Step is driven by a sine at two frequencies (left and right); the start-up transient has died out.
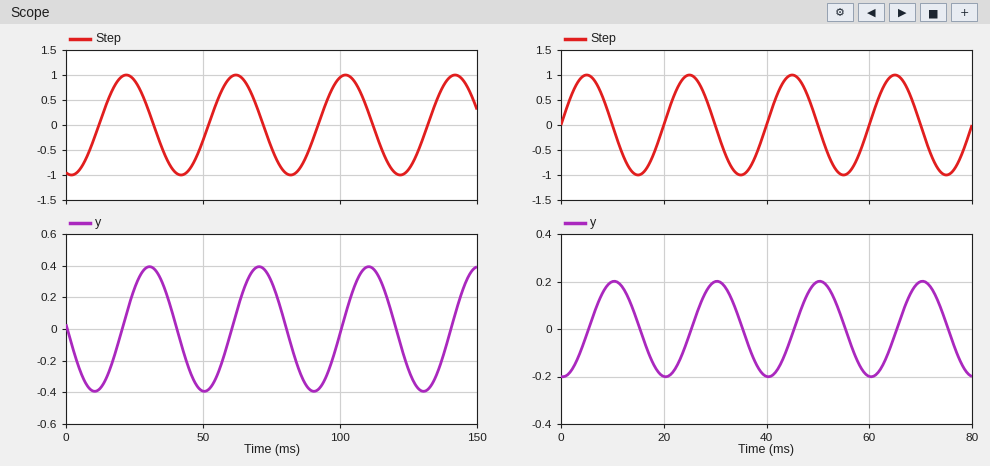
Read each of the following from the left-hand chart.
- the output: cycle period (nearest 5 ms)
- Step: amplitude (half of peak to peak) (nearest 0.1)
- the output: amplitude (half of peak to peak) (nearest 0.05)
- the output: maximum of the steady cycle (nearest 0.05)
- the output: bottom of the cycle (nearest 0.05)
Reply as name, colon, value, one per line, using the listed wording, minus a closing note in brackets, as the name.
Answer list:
the output: cycle period: 40 ms
Step: amplitude (half of peak to peak): 1.0
the output: amplitude (half of peak to peak): 0.40
the output: maximum of the steady cycle: 0.40
the output: bottom of the cycle: -0.40
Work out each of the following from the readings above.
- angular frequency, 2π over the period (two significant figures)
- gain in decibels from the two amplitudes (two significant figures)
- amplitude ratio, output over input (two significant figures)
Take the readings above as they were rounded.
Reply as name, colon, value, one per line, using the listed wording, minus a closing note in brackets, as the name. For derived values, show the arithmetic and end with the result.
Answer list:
angular frequency, 2π over the period: 2π / 40 = 0.16 rad/ms
gain in decibels from the two amplitudes: 20 log10(0.4 / 1) = -8.0 dB
amplitude ratio, output over input: 0.4 / 1 = 0.40
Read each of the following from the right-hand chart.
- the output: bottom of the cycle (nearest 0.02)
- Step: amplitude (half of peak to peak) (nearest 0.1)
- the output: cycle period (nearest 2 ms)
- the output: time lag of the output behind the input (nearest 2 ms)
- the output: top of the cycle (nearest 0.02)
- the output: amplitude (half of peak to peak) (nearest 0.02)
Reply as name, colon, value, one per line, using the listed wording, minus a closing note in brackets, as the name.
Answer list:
the output: bottom of the cycle: -0.20
Step: amplitude (half of peak to peak): 1.0
the output: cycle period: 20 ms
the output: time lag of the output behind the input: 6 ms
the output: top of the cycle: 0.20
the output: amplitude (half of peak to peak): 0.20
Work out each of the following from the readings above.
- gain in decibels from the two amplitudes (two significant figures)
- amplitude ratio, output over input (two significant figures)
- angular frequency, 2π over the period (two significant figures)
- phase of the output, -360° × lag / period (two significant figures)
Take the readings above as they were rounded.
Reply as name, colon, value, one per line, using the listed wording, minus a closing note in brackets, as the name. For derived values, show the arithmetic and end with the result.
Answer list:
gain in decibels from the two amplitudes: 20 log10(0.2 / 1) = -14 dB
amplitude ratio, output over input: 0.2 / 1 = 0.20
angular frequency, 2π over the period: 2π / 20 = 0.31 rad/ms
phase of the output, -360° × lag / period: -360 × 6 / 20 = -110°
